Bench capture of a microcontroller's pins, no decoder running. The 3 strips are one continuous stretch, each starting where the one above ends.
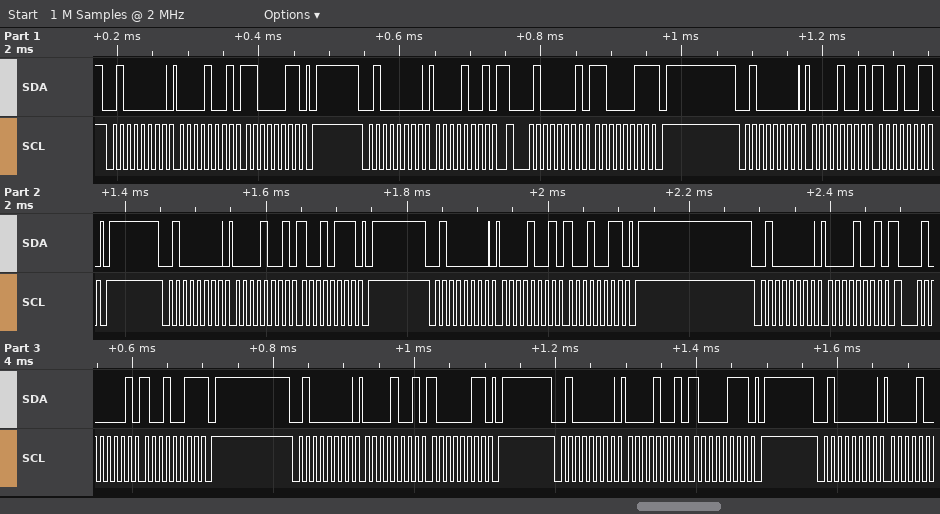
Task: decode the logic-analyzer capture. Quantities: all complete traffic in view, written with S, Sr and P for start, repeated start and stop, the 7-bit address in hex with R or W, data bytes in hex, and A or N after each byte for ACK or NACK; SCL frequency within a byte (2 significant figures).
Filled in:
S 20W A 09 A C3 A P S 20W A 09 A Sr 20R A C3 N P S 20W A 09 A 93 A P S 20W A 09 A 97 A P S 20W A 09 A 93 A P S 20W A 09 A Sr 20R A 93 N P S 20W A 09 A 83 A P S 20W A 09 A 87 A P S 20W A
100 kHz
